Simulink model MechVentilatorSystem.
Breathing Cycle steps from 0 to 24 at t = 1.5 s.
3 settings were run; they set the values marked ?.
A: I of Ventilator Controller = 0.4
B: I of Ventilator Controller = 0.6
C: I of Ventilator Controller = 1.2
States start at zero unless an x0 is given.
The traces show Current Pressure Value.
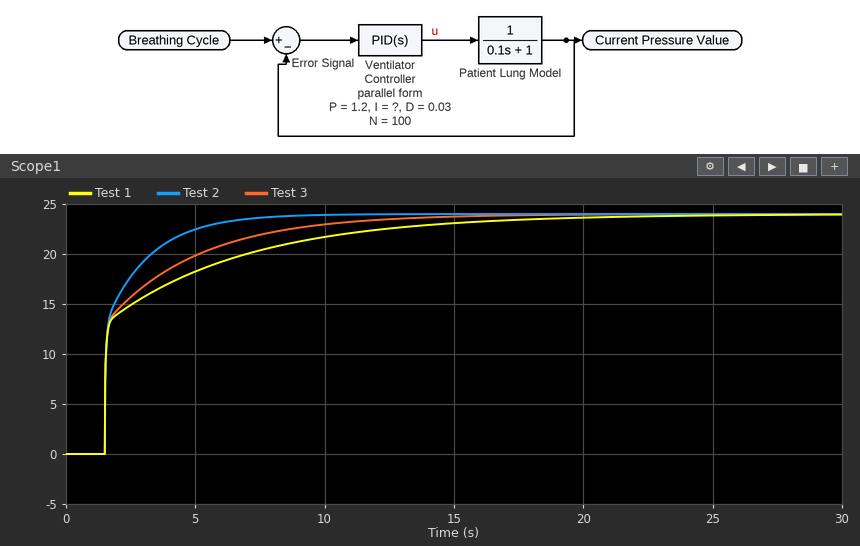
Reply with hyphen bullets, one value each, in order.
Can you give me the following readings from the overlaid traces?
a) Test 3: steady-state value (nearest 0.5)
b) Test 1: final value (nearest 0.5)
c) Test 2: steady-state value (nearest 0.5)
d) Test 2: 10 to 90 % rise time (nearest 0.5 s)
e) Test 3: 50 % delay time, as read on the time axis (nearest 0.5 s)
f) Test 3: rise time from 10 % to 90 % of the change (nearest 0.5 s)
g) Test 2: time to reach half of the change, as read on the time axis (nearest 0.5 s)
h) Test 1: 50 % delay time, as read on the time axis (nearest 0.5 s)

- 24.0
- 24.0
- 24.0
- 2.5 s
- 1.5 s
- 5.5 s
- 1.5 s
- 1.5 s
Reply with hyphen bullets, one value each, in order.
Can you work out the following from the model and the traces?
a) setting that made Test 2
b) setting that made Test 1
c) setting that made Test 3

- C
- A
- B
